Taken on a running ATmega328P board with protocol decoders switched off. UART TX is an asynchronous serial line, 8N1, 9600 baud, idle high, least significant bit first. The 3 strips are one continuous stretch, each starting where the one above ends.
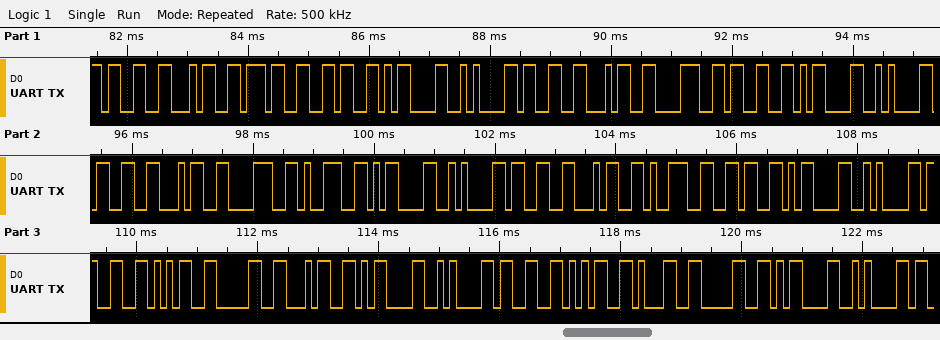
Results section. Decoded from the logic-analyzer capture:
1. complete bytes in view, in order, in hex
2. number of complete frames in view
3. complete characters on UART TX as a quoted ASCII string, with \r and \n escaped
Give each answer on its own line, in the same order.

33 34 37 36 0D 0A 33 34 38 33 0D 0A 33 34 38 39 0D 0A 33 34 39 36 0D 0A 33 35 30 34 0D 0A 33 35 31 30 0D 0A
36
"3476\r\n3483\r\n3489\r\n3496\r\n3504\r\n3510\r\n"
